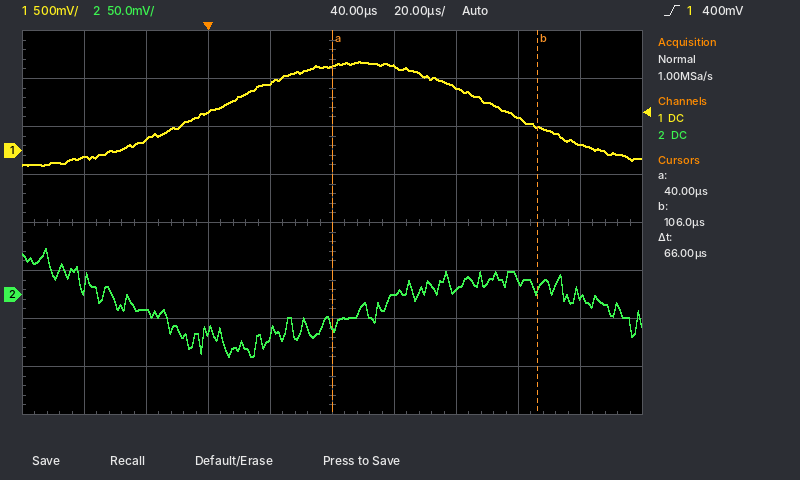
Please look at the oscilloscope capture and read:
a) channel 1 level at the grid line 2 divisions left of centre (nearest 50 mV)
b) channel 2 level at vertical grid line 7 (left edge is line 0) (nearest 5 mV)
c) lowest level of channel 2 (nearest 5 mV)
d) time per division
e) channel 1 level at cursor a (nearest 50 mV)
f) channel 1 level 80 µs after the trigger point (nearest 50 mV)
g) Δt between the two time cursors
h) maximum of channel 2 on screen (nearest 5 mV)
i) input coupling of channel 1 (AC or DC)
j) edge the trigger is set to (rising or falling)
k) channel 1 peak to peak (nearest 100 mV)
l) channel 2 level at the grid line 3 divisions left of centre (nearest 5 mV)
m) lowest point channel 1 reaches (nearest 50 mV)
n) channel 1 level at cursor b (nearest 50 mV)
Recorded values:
400 mV
5 mV
-65 mV
20 µs
900 mV
650 mV
66 µs
50 mV
DC
rising
1.10 V
-15 mV
-150 mV
250 mV
